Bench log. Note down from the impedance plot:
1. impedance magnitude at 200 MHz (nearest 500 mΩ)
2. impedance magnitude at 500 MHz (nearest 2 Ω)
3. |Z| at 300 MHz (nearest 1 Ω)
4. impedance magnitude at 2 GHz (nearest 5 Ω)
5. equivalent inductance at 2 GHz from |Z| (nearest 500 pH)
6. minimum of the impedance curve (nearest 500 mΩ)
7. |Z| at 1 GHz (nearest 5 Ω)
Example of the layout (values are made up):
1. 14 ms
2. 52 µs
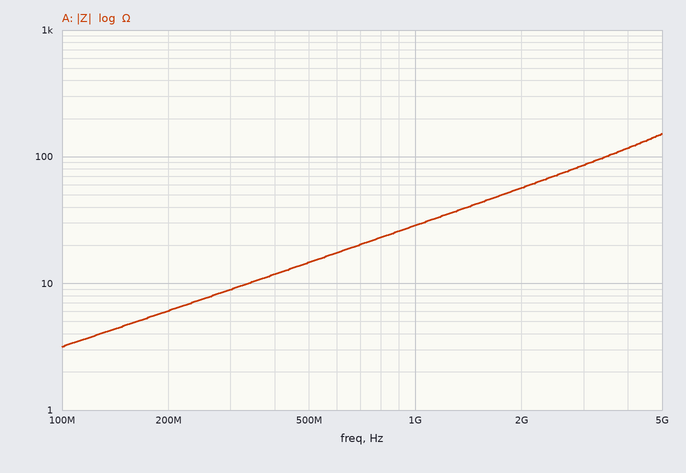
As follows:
1. 6.0 Ω
2. 14 Ω
3. 9 Ω
4. 55 Ω
5. 4.5 nH
6. 3.0 Ω
7. 30 Ω
